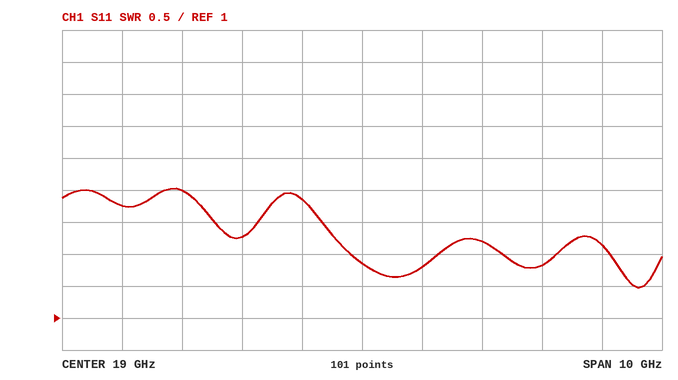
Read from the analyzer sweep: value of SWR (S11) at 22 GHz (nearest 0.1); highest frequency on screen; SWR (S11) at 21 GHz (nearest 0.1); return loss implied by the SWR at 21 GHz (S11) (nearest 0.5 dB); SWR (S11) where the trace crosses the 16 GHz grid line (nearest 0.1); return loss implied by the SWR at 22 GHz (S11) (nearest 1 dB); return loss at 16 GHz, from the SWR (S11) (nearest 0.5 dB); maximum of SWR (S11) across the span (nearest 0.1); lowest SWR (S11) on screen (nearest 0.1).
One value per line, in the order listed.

1.8
24 GHz
2.2
8.5 dB
3.0
11 dB
6.0 dB
3.0
1.5
